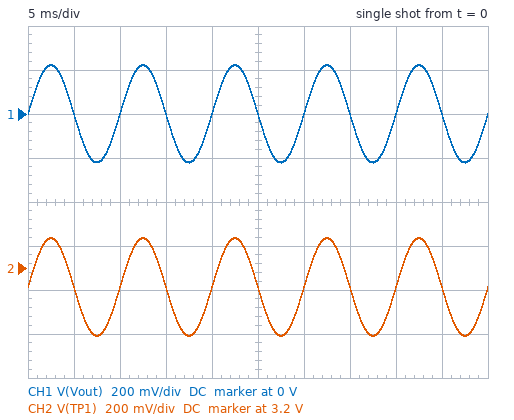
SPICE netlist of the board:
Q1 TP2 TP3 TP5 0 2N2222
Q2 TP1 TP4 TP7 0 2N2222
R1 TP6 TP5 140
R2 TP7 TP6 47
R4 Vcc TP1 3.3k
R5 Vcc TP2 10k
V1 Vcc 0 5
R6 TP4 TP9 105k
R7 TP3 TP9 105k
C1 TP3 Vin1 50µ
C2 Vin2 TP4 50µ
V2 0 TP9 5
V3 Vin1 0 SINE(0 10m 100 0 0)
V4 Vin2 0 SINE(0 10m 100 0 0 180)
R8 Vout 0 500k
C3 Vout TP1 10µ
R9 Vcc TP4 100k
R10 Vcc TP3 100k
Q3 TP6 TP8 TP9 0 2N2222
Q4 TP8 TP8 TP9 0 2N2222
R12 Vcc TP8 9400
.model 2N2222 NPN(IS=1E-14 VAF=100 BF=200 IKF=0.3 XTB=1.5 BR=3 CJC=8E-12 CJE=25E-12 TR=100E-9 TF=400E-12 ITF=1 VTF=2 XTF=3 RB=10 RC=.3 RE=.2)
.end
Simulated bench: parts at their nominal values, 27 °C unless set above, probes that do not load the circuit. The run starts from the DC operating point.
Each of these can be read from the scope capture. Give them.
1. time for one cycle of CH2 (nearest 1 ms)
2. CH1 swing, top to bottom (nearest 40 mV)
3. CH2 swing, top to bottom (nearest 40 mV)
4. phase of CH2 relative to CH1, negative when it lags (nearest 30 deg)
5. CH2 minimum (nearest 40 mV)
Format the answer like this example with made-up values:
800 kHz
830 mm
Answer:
10 ms
440 mV
440 mV
0 deg
2.88 V
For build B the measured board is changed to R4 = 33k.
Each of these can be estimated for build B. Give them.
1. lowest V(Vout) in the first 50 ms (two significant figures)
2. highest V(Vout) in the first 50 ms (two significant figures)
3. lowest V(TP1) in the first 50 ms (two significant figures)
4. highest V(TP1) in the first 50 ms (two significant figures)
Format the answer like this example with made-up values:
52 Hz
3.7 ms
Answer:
-9.5 mV
42 mV
-2.3 V
-2.2 V
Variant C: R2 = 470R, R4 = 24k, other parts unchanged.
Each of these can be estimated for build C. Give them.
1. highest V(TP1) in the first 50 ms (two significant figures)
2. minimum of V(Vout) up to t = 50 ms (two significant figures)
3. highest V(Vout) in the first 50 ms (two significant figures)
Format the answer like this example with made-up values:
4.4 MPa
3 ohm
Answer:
-1.7 V
-6.4 mV
27 mV
